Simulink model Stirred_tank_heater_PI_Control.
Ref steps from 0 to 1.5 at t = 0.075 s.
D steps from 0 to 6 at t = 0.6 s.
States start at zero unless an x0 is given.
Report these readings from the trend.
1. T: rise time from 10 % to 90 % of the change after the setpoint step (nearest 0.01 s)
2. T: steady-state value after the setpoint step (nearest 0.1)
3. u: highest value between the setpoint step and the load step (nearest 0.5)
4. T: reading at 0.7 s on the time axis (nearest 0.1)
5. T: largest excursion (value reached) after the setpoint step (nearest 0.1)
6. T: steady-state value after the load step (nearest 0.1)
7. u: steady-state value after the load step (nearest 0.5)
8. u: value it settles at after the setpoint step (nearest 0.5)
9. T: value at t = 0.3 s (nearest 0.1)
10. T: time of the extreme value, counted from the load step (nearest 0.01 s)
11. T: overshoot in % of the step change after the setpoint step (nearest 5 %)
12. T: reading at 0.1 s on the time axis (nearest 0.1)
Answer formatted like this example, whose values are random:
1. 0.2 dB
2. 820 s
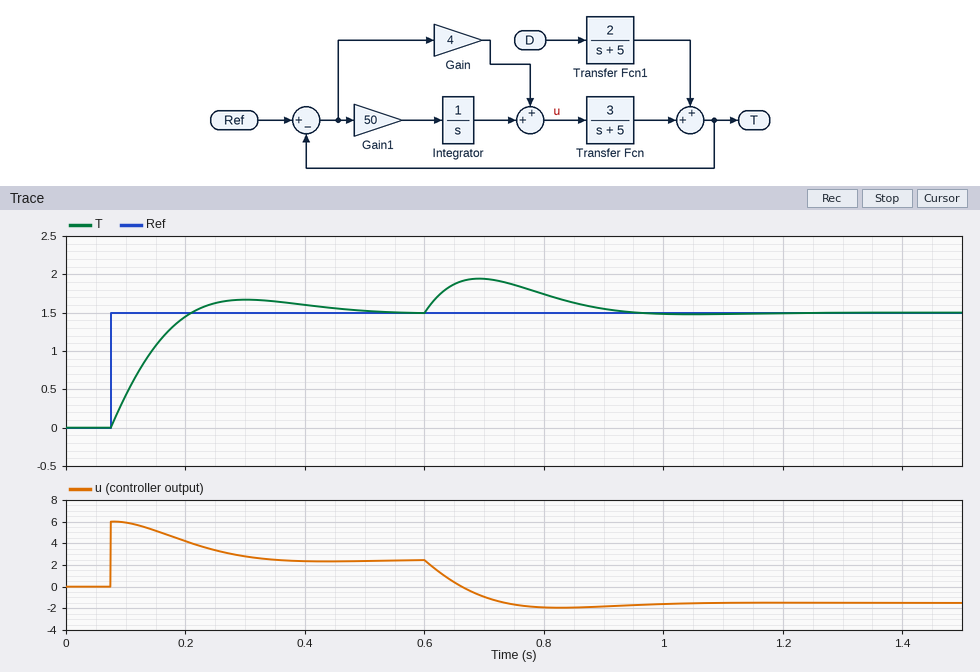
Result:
1. 0.10 s
2. 1.5
3. 6.0
4. 1.9
5. 1.7
6. 1.5
7. -1.5
8. 2.5
9. 1.7
10. 0.09 s
11. 10 %
12. 0.4
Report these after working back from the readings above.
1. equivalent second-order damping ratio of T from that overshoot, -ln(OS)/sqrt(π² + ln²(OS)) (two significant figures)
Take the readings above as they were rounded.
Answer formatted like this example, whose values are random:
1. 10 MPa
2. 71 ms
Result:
1. 0.59
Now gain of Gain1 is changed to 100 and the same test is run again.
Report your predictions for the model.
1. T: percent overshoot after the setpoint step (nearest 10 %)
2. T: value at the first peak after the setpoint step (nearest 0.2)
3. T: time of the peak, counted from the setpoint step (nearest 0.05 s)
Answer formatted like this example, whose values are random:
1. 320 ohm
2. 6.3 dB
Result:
1. 20 %
2. 1.8
3. 0.15 s
